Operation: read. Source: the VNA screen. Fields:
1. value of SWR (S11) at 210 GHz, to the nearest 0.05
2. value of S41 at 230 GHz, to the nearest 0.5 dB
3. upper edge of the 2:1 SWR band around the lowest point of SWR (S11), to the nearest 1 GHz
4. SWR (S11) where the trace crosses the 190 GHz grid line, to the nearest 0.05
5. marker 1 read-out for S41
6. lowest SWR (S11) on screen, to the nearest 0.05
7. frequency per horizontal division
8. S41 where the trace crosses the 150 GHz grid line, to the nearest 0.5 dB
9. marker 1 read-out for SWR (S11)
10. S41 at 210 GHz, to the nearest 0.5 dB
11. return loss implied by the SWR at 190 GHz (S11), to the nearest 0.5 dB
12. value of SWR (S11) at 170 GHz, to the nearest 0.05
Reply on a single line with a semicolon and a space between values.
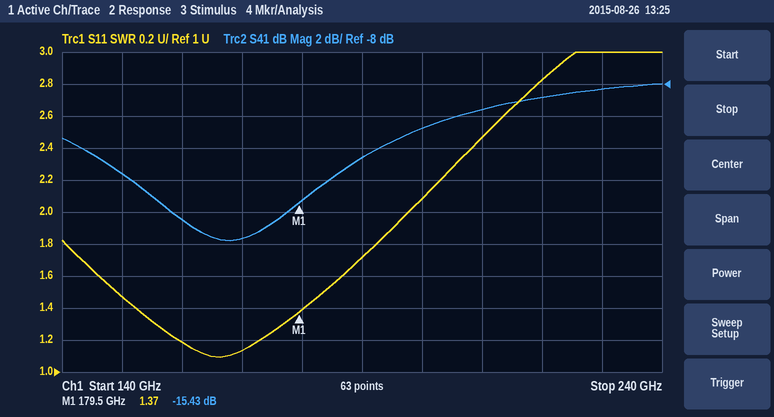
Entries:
2.45; -8.5 dB; 198 GHz; 1.70; -15.43 dB; 1.10; 10 GHz; -13.5 dB; 1.37; -9.5 dB; 11.5 dB; 1.15
